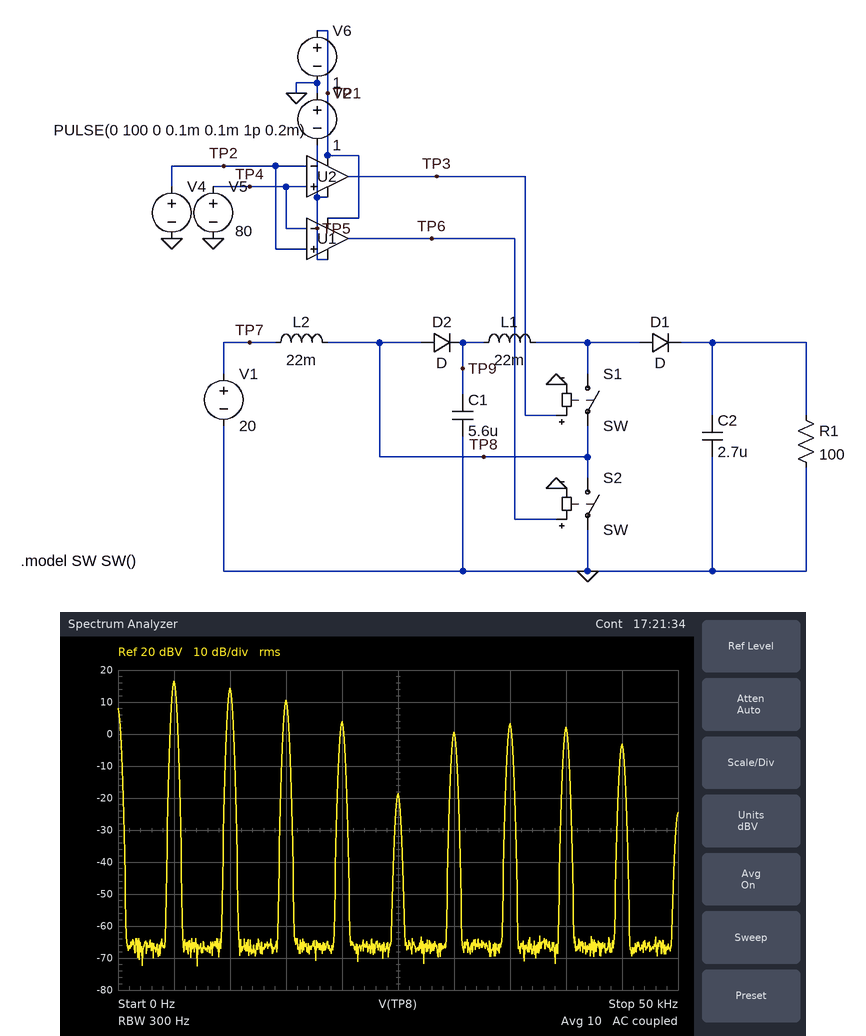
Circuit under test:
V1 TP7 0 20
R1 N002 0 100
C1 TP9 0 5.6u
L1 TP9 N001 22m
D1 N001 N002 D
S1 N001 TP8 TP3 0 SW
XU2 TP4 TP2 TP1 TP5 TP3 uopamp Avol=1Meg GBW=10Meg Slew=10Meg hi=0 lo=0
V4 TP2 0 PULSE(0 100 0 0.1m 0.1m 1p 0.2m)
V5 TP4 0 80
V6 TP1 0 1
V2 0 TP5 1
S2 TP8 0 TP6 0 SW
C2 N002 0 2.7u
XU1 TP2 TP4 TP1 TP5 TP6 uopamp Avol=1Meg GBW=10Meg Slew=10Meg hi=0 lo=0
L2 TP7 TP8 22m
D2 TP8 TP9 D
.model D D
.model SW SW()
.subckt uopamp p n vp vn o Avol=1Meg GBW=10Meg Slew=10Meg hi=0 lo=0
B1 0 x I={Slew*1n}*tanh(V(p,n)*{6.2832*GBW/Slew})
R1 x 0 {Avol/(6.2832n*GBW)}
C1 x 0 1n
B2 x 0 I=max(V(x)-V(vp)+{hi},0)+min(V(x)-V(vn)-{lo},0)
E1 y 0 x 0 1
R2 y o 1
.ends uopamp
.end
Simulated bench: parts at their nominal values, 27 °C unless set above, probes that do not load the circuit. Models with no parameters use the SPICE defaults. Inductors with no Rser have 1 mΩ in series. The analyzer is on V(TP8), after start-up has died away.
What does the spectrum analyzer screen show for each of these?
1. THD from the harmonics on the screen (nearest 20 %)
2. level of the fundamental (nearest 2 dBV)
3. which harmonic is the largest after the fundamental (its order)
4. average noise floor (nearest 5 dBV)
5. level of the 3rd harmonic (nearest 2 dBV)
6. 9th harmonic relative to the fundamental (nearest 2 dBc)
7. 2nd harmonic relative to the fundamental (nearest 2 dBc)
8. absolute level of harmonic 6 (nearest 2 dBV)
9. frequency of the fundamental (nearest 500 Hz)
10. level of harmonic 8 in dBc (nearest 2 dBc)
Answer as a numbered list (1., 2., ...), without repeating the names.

1. 100 %
2. 16 dBV
3. 2
4. -65 dBV
5. 10 dBV
6. -20 dBc
7. -2 dBc
8. 0 dBV
9. 5.0 kHz
10. -14 dBc
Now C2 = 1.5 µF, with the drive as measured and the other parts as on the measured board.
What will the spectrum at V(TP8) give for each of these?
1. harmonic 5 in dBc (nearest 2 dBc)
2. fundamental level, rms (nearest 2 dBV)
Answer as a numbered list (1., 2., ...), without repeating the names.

1. -30 dBc
2. 16 dBV
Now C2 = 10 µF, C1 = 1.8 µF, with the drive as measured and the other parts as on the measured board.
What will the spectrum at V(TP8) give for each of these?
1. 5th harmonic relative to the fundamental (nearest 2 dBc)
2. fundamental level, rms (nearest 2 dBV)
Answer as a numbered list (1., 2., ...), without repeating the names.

1. -44 dBc
2. 16 dBV
